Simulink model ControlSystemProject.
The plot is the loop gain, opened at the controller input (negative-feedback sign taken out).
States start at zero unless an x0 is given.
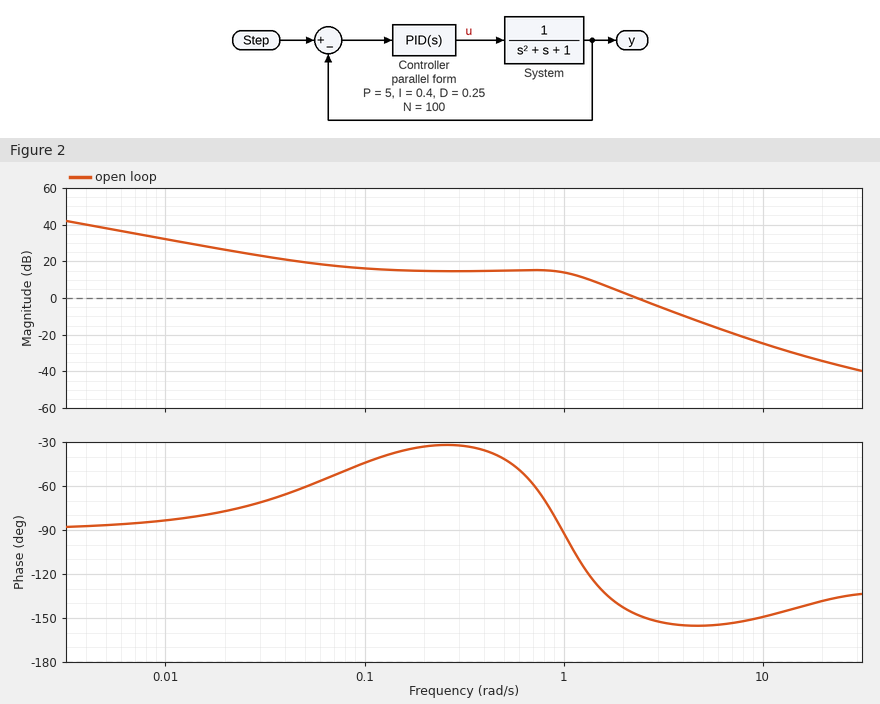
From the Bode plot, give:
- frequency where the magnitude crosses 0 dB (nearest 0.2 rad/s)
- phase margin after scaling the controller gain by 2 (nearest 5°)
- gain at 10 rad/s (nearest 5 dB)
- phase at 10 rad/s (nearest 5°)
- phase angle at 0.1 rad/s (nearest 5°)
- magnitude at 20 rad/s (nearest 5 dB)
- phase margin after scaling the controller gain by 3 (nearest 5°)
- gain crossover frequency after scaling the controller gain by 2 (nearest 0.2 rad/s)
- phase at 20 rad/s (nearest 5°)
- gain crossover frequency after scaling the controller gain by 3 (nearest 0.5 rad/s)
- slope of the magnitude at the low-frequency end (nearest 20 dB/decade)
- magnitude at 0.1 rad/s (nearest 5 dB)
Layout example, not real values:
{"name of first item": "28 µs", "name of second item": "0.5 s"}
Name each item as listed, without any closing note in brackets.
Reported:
{"frequency where the magnitude crosses 0 dB": "2.4 rad/s", "phase margin after scaling the controller gain by 2": "25°", "gain at 10 rad/s": "-25 dB", "phase at 10 rad/s": "-150°", "phase angle at 0.1 rad/s": "-45°", "magnitude at 20 rad/s": "-35 dB", "phase margin after scaling the controller gain by 3": "25°", "gain crossover frequency after scaling the controller gain by 2": "3.2 rad/s", "phase at 20 rad/s": "-140°", "gain crossover frequency after scaling the controller gain by 3": "4.0 rad/s", "slope of the magnitude at the low-frequency end": "-20 dB/decade", "magnitude at 0.1 rad/s": "15 dB"}
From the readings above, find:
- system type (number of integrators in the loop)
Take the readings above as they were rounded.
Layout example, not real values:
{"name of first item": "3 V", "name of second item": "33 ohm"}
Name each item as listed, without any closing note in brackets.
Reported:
{"system type": "1"}
